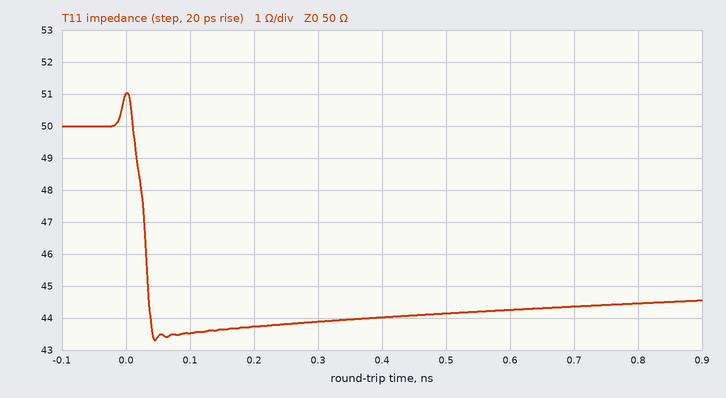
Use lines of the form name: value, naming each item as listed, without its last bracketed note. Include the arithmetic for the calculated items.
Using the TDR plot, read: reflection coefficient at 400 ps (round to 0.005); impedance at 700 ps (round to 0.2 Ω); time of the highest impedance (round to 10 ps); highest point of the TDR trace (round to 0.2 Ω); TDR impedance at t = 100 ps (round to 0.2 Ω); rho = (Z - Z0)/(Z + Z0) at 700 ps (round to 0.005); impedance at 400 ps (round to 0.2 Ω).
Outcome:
reflection coefficient at 400 ps: (44 − 50)/(44 + 50) ≈ -0.0638, so -0.065 to the nearest 0.005
impedance at 700 ps: 44.4 Ω
time of the highest impedance: 0 ps
highest point of the TDR trace: 51.0 Ω
TDR impedance at t = 100 ps: 43.6 Ω
rho = (Z - Z0)/(Z + Z0) at 700 ps: (44.4 − 50)/(44.4 + 50) ≈ -0.0593, so -0.060 to the nearest 0.005
impedance at 400 ps: 44.0 Ω
